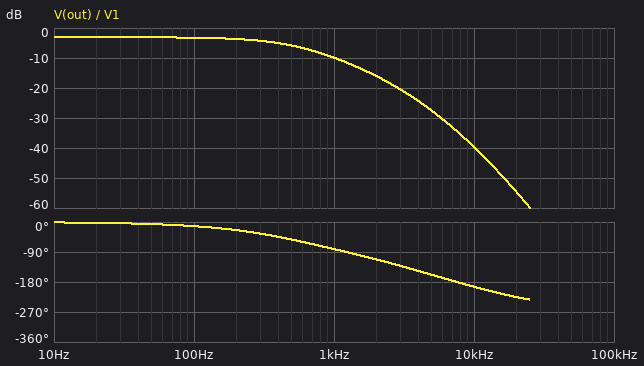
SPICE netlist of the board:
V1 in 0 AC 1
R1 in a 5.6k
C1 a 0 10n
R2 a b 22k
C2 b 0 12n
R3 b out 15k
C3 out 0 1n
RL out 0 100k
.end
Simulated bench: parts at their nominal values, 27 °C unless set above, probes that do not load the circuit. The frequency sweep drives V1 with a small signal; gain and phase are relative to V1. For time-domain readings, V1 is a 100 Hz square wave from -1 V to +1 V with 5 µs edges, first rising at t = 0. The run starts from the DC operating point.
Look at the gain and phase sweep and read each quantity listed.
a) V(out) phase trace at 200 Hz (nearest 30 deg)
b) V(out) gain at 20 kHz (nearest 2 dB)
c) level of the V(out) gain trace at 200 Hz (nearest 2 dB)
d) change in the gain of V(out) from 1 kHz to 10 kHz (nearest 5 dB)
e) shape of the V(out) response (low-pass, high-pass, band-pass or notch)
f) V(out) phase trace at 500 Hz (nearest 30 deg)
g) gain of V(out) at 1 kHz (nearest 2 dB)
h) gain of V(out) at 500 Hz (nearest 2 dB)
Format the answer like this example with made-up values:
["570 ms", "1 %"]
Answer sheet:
["-30 deg", "-54 dB", "-4 dB", "-30 dB", "low-pass", "-60 deg", "-10 dB", "-6 dB"]
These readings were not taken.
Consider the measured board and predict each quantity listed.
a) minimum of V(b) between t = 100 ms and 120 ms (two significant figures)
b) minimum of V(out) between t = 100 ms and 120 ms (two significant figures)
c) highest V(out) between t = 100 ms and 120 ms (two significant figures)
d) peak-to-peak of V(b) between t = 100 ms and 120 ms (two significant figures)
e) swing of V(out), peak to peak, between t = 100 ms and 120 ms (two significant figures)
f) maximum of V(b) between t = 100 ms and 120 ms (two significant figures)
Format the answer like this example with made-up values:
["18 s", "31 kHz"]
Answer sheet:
["-810 mV", "-700 mV", "700 mV", "1.6 V", "1.4 V", "810 mV"]
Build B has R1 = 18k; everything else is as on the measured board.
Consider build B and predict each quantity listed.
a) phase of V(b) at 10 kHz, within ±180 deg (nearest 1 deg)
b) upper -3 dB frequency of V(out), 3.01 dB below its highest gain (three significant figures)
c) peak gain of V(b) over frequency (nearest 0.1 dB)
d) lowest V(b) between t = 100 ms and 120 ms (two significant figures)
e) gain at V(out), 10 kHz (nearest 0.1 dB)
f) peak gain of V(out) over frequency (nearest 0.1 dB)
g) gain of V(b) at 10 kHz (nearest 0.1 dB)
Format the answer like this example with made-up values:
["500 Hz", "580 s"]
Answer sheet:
["-165 deg", "338 Hz", "-2.6 dB", "-740 mV", "-49.4 dB", "-3.8 dB", "-46.0 dB"]
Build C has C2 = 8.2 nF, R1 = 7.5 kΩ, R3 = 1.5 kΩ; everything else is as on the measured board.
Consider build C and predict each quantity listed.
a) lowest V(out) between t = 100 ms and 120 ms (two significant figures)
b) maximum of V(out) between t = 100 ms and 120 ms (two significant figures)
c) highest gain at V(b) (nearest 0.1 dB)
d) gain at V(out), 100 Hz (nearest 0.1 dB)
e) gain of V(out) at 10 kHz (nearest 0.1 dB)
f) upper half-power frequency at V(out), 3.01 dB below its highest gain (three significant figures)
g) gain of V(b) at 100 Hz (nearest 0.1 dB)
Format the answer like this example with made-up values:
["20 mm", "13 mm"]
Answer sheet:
["-760 mV", "760 mV", "-2.2 dB", "-2.4 dB", "-36.1 dB", "663 Hz", "-2.3 dB"]
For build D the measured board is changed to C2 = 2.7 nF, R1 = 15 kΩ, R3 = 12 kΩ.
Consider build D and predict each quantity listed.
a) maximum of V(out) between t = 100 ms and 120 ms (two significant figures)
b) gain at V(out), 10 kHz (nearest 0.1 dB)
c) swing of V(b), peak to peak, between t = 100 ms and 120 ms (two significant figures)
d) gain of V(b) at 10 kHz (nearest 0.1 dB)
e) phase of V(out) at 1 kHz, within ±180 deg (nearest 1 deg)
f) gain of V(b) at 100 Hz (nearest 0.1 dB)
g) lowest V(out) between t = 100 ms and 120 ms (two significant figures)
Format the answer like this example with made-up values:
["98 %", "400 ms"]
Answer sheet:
["670 mV", "-36.0 dB", "1.5 V", "-33.4 dB", "-69 deg", "-2.5 dB", "-670 mV"]
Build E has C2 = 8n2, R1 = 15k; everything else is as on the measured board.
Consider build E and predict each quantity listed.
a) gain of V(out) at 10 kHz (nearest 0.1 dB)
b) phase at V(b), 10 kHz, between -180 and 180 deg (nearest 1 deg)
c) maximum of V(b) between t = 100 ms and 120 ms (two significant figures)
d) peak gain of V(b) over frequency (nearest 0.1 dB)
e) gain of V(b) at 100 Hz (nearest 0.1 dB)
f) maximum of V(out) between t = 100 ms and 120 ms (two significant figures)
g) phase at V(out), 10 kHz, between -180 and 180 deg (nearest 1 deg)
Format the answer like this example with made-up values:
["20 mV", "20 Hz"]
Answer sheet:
["-44.8 dB", "-162 deg", "760 mV", "-2.4 dB", "-2.6 dB", "660 mV", "159 deg"]
